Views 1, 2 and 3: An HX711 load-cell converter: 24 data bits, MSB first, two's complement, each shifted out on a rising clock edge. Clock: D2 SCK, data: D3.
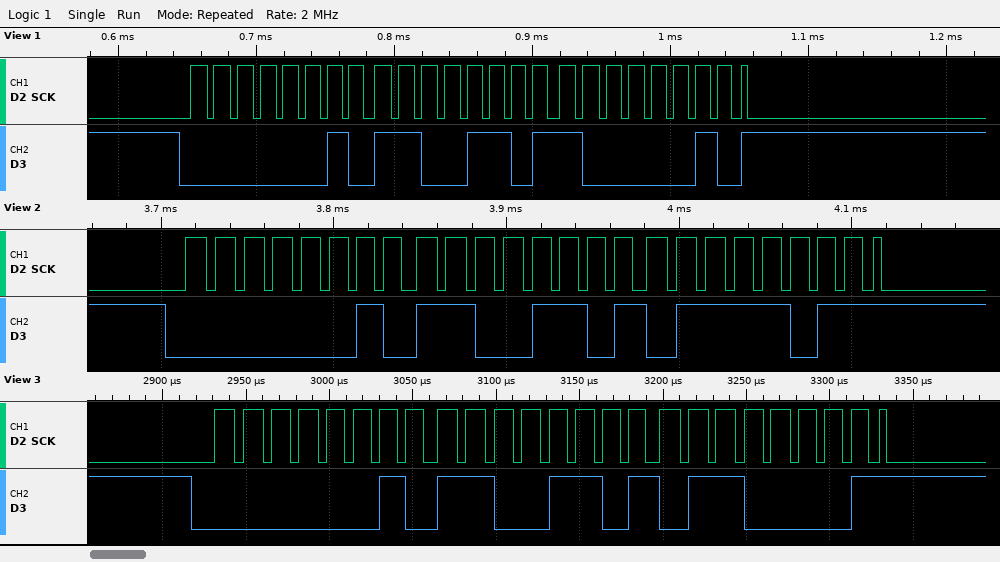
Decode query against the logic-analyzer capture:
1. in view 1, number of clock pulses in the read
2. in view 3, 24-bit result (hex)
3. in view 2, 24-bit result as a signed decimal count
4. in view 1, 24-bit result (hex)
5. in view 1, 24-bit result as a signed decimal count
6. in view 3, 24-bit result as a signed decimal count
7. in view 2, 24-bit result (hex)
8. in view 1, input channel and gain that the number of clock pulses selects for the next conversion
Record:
25
0x02CD61
183675
0x02CD82
183682
183649
0x02CD7B
channel A, gain 128
